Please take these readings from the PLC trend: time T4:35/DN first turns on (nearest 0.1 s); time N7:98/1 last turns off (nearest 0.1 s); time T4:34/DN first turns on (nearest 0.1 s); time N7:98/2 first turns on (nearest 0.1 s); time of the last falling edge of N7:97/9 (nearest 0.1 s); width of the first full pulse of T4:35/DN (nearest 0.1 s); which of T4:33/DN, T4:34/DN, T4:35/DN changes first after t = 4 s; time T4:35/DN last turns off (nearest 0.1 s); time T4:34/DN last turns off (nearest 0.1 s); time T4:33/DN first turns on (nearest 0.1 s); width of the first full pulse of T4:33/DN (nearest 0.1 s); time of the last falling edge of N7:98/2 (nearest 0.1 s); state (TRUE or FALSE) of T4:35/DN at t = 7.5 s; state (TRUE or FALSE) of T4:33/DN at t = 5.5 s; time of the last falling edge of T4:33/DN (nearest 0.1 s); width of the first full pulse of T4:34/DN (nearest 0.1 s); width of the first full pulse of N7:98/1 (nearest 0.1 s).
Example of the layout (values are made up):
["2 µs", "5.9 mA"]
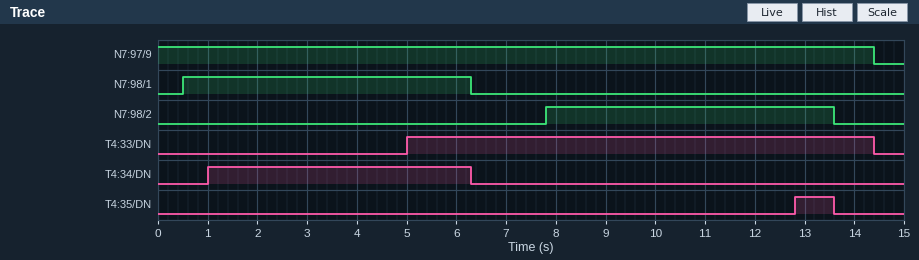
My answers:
["12.8 s", "6.3 s", "1.0 s", "7.8 s", "14.4 s", "0.8 s", "T4:33/DN", "13.6 s", "6.3 s", "5.0 s", "9.4 s", "13.6 s", "FALSE", "TRUE", "14.4 s", "5.3 s", "5.8 s"]
